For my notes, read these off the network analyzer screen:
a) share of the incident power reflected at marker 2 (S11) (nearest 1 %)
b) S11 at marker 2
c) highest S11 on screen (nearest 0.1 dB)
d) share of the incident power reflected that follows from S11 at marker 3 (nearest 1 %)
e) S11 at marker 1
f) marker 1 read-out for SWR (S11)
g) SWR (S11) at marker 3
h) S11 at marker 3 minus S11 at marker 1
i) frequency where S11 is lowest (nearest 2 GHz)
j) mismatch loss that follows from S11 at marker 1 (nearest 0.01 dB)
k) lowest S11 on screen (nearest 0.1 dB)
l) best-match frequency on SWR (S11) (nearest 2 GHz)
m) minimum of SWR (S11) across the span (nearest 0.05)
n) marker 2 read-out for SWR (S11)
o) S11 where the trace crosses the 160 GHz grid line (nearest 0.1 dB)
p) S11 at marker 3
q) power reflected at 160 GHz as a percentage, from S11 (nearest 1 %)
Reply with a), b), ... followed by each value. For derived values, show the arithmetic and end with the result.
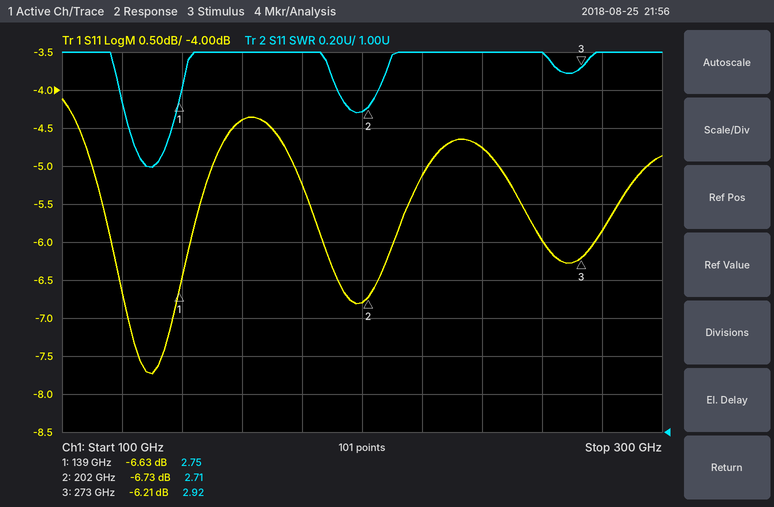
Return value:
a) 10^(-6.73/10) ≈ 21 %
b) -6.73 dB
c) -4.1 dB
d) 10^(-6.21/10) ≈ 24 %
e) -6.63 dB
f) 2.75
g) 2.92
h) -6.21 − (-6.63) = 0.42 dB
i) 130 GHz
j) −10 log10(1 − 10^(-6.63/10)) ≈ 1.06 dB
k) -7.7 dB
l) 130 GHz
m) 2.40
n) 2.71
o) -4.4 dB
p) -6.21 dB
q) 10^(-4.4/10) ≈ 36 %
